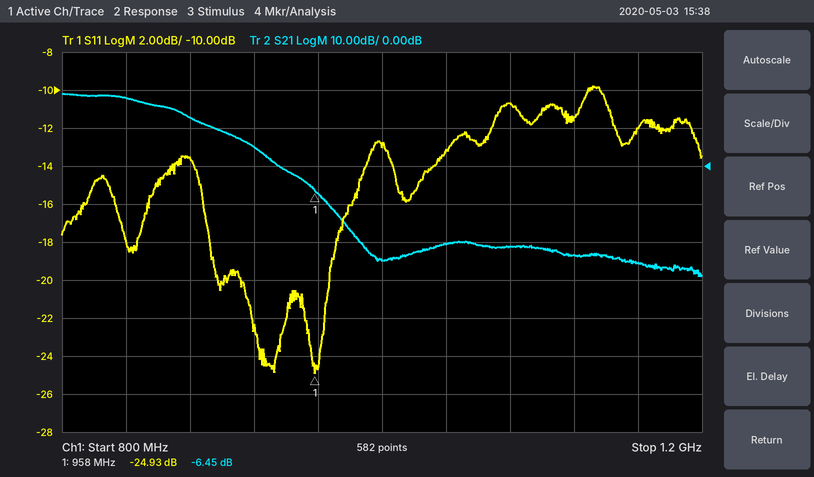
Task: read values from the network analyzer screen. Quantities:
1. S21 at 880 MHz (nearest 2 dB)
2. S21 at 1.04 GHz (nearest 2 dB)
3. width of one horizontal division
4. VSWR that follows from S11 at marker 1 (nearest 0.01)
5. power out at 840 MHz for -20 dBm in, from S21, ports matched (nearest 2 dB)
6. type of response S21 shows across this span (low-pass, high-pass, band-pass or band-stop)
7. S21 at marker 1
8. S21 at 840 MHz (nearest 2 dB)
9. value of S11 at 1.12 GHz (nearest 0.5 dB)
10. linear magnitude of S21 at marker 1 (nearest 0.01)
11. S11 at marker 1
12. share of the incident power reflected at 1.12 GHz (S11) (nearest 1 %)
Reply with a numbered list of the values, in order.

1. 12 dB
2. -20 dB
3. 40 MHz
4. 1.12
5. -2 dBm
6. low-pass
7. -6.45 dB
8. 18 dB
9. -11.5 dB
10. 0.48
11. -24.93 dB
12. 7 %
